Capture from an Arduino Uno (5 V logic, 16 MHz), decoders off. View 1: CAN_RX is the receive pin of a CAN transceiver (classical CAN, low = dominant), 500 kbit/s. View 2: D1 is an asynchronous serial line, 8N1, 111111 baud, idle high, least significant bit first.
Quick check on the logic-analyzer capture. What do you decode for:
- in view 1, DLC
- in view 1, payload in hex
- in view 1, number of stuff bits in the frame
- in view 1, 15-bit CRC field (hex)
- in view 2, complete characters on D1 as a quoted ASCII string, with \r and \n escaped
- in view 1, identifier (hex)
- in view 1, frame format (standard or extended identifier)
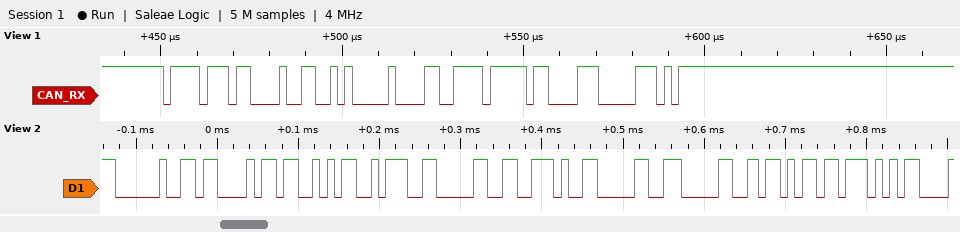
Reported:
4
CA 00 CF 7F
3
0x0706
" CS:0.00kW"
0x7BB
standard
